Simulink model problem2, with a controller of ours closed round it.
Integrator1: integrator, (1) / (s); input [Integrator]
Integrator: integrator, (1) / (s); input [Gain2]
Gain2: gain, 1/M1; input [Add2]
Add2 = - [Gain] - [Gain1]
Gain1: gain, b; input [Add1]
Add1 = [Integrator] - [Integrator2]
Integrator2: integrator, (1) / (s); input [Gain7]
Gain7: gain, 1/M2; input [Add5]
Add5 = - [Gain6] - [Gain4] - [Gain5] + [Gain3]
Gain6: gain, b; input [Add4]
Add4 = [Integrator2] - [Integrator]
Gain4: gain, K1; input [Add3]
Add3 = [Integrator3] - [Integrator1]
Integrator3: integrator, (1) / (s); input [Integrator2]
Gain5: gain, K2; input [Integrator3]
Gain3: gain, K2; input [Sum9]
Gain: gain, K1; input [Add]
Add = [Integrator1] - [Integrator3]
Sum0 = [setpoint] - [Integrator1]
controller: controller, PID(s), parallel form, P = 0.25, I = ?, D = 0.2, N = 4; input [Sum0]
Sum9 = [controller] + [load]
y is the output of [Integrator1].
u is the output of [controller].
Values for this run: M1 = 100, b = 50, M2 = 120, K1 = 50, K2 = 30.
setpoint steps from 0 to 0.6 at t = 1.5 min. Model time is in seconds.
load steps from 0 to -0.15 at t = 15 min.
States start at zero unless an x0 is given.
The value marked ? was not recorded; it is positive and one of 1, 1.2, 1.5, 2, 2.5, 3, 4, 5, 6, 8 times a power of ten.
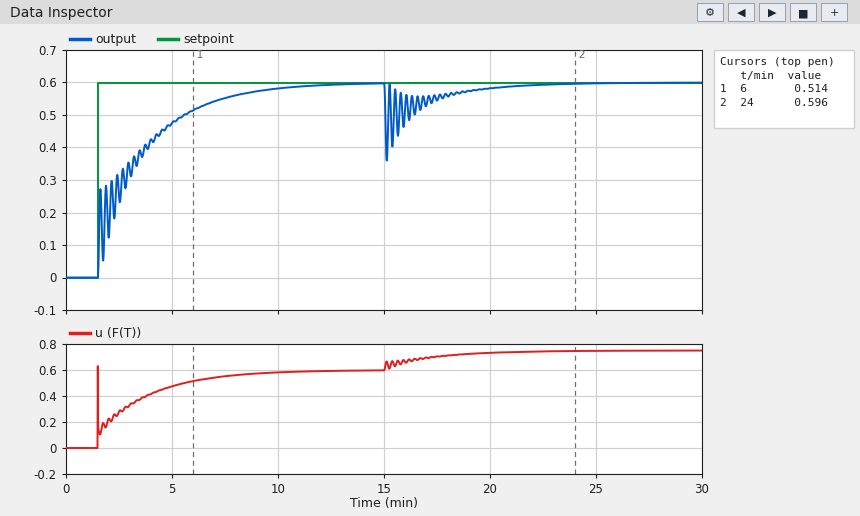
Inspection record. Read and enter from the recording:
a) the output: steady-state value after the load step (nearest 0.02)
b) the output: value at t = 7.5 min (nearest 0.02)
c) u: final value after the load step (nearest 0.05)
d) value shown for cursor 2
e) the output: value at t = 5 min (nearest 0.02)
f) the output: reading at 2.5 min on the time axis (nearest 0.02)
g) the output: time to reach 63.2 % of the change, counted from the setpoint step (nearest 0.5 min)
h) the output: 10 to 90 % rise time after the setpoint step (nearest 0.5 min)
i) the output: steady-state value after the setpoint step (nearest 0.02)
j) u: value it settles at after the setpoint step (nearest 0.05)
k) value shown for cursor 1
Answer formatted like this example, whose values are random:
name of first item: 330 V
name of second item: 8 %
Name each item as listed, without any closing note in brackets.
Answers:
the output: steady-state value after the load step: 0.60
the output: value at t = 7.5 min: 0.56
u: final value after the load step: 0.75
value shown for cursor 2: 0.596
the output: value at t = 5 min: 0.48
the output: reading at 2.5 min on the time axis: 0.26
the output: time to reach 63.2 % of the change, counted from the setpoint step: 2.0 min
the output: 10 to 90 % rise time after the setpoint step: 5.5 min
the output: steady-state value after the setpoint step: 0.60
u: value it settles at after the setpoint step: 0.60
value shown for cursor 1: 0.514
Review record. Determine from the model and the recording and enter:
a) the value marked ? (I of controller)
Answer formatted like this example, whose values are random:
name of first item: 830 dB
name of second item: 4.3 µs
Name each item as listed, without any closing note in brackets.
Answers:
the value marked ?: 0.008
